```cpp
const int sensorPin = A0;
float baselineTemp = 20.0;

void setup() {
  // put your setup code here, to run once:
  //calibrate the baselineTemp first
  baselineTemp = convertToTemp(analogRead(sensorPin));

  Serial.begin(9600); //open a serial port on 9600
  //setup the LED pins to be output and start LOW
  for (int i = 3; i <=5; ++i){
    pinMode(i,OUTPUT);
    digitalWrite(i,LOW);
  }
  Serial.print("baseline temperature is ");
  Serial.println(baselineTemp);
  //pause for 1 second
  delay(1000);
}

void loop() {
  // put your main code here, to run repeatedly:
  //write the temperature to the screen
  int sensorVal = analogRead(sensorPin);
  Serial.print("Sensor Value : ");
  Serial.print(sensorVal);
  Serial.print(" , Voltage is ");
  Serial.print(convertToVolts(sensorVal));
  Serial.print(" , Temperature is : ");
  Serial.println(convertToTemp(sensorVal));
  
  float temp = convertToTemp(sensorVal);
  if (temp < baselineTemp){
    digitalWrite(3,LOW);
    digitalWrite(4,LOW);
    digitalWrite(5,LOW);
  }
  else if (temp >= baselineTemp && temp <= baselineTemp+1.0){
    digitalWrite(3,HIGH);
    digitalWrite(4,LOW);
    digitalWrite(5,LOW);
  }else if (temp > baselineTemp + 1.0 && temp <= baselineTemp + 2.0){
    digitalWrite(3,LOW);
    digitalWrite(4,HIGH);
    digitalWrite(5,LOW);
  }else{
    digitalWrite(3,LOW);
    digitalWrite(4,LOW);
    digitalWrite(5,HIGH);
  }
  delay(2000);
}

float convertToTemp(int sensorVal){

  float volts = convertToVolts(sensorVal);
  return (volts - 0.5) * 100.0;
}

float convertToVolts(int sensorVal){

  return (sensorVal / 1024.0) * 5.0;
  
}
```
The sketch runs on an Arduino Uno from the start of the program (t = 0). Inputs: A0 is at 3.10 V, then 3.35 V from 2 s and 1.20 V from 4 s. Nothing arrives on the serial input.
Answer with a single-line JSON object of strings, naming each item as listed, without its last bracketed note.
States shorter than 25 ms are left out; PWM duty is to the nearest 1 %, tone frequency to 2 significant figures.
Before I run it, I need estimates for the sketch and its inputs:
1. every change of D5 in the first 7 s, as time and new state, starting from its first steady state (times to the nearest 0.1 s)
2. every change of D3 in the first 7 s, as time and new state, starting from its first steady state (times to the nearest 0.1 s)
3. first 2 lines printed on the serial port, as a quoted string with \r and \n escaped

{"every change of D5 in the first 7 s, as time and new state, starting from its first steady state": "0 s low; 3 s high; 5 s low", "every change of D3 in the first 7 s, as time and new state, starting from its first steady state": "0 s low; 1 s high; 3 s low", "first 2 lines printed on the serial port, as a quoted string with \\r and \\n escaped": "\"baseline temperature is 259.57\\r\\nSensor Value : 634 , Voltage is 3.10 , Temperature is : 259.57\\r\\n\""}
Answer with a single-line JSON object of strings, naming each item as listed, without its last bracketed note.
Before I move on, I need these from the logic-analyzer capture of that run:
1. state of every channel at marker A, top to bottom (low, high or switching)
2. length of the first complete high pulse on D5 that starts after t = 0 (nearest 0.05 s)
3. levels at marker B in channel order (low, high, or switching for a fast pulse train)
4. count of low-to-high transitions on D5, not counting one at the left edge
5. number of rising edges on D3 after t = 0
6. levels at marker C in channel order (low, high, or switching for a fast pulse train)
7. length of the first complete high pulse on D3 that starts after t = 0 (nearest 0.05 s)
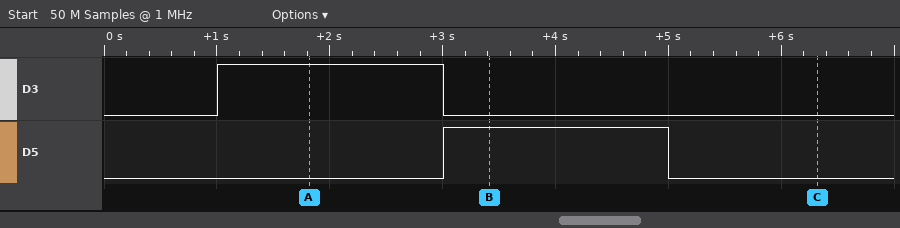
{"state of every channel at marker A, top to bottom": "D3 high, D5 low", "length of the first complete high pulse on D5 that starts after t = 0": "2.00 s", "levels at marker B in channel order": "D3 low, D5 high", "count of low-to-high transitions on D5, not counting one at the left edge": "1", "number of rising edges on D3 after t = 0": "1", "levels at marker C in channel order": "D3 low, D5 low", "length of the first complete high pulse on D3 that starts after t = 0": "2.00 s"}
